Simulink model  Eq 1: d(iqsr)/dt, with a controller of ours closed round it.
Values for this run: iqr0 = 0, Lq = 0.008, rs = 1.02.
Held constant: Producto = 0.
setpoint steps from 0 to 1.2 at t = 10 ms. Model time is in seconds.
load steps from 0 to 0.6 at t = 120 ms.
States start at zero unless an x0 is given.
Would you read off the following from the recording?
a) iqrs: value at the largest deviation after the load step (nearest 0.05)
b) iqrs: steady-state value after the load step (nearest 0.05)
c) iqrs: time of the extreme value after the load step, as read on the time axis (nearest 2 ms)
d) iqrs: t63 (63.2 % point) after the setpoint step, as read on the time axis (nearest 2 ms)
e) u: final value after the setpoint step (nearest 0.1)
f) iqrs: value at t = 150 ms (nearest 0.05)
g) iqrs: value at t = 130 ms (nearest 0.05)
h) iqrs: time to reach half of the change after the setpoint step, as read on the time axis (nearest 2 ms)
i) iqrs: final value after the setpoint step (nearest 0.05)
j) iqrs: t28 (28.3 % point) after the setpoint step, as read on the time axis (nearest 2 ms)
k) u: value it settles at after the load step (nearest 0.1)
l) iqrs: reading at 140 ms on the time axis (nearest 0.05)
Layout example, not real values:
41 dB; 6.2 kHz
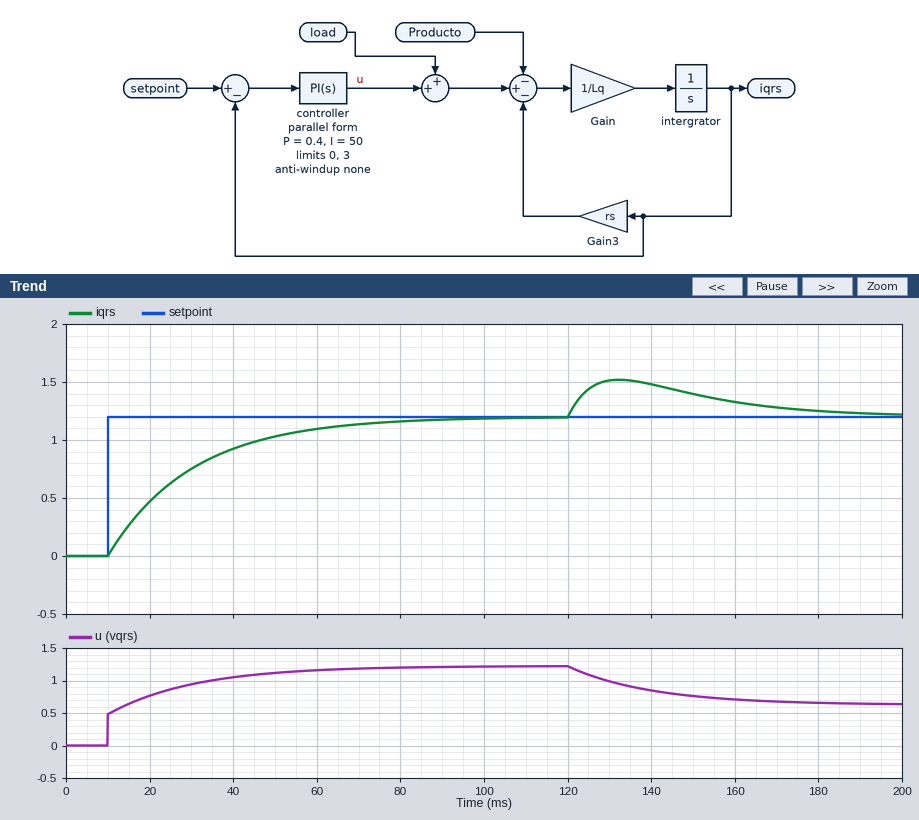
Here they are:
1.50; 1.20; 132 ms; 30 ms; 1.2; 1.40; 1.50; 24 ms; 1.20; 16 ms; 0.6; 1.50
